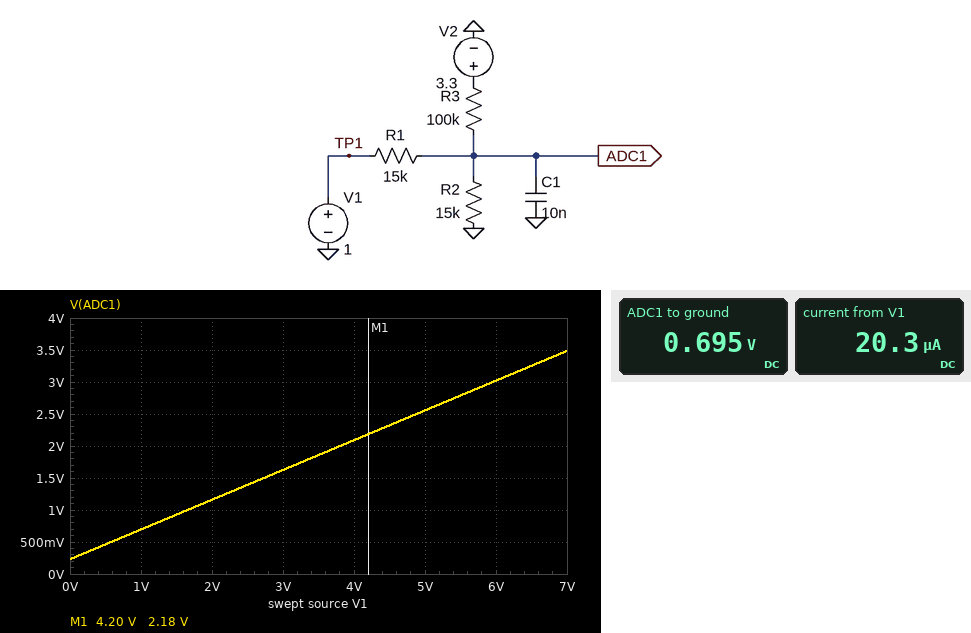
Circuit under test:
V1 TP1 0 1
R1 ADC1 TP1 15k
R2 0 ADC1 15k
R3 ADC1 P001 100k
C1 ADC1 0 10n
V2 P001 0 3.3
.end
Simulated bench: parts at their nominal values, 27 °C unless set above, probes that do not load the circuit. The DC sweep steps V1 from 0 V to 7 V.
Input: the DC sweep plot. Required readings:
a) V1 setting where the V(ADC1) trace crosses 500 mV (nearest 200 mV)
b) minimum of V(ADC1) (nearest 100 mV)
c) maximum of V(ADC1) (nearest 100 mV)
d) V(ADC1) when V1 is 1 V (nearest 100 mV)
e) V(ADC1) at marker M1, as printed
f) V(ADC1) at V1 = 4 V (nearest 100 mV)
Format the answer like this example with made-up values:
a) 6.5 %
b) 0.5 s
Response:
a) 600 mV
b) 200 mV
c) 3.5 V
d) 700 mV
e) 2.18 V
f) 2.1 V
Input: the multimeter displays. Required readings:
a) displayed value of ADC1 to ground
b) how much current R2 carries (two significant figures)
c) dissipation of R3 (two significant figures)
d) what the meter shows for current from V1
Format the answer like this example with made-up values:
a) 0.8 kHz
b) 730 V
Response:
a) 0.695 V
b) 46 µA
c) 68 µW
d) 20.3 µA
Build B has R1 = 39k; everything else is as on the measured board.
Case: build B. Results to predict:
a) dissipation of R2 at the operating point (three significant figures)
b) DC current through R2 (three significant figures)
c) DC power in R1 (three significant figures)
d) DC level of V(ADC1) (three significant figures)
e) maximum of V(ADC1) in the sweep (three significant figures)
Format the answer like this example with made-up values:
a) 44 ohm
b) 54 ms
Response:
a) 21.9 µW
b) 38.2 µA
c) 4.67 µW
d) 573 mV
e) 2.08 V
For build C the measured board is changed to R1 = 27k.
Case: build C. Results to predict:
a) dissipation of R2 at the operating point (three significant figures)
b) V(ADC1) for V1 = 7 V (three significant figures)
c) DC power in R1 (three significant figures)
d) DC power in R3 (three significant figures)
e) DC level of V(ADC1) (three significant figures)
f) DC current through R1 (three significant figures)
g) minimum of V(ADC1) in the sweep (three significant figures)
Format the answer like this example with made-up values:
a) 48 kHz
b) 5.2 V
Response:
a) 25.3 µW
b) 2.57 V
c) 5.46 µW
d) 72.0 µW
e) 616 mV
f) 14.2 µA
g) 290 mV
